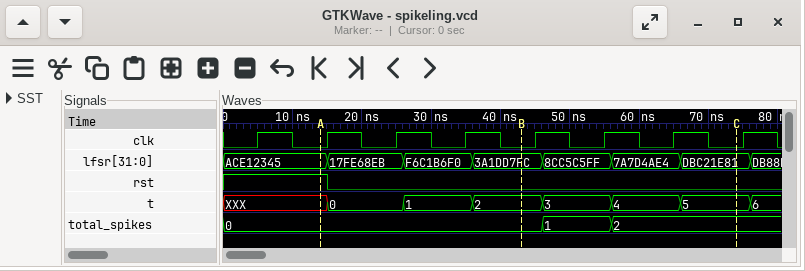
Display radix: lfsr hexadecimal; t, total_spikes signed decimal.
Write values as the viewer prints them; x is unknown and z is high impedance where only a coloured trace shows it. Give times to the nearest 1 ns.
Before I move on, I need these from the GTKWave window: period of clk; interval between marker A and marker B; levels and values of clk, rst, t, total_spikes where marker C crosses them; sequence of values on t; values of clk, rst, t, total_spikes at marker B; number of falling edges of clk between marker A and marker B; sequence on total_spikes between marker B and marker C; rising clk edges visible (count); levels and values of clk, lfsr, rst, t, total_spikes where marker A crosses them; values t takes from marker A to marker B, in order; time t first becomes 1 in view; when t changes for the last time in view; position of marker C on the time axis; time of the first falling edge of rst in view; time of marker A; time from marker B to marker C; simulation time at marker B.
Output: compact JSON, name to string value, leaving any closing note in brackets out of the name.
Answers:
{"period of clk": "10 ns", "interval between marker A and marker B": "29 ns", "levels and values of clk, rst, t, total_spikes where marker C crosses them": "clk=0, rst=0, t=5, total_spikes=2", "sequence of values on t": "XXX, 0, 1, 2, 3, 4, 5, 6", "values of clk, rst, t, total_spikes at marker B": "clk=0, rst=0, t=2, total_spikes=0", "number of falling edges of clk between marker A and marker B": "3", "sequence on total_spikes between marker B and marker C": "0, 1, 2", "rising clk edges visible": "8", "levels and values of clk, lfsr, rst, t, total_spikes where marker A crosses them": "clk=0, lfsr=ACE12345, rst=1, t=XXX, total_spikes=0", "values t takes from marker A to marker B, in order": "XXX, 0, 1, 2", "time t first becomes 1 in view": "26 ns", "when t changes for the last time in view": "76 ns", "position of marker C on the time axis": "74 ns", "time of the first falling edge of rst in view": "15 ns", "time of marker A": "14 ns", "time from marker B to marker C": "31 ns", "simulation time at marker B": "43 ns"}
